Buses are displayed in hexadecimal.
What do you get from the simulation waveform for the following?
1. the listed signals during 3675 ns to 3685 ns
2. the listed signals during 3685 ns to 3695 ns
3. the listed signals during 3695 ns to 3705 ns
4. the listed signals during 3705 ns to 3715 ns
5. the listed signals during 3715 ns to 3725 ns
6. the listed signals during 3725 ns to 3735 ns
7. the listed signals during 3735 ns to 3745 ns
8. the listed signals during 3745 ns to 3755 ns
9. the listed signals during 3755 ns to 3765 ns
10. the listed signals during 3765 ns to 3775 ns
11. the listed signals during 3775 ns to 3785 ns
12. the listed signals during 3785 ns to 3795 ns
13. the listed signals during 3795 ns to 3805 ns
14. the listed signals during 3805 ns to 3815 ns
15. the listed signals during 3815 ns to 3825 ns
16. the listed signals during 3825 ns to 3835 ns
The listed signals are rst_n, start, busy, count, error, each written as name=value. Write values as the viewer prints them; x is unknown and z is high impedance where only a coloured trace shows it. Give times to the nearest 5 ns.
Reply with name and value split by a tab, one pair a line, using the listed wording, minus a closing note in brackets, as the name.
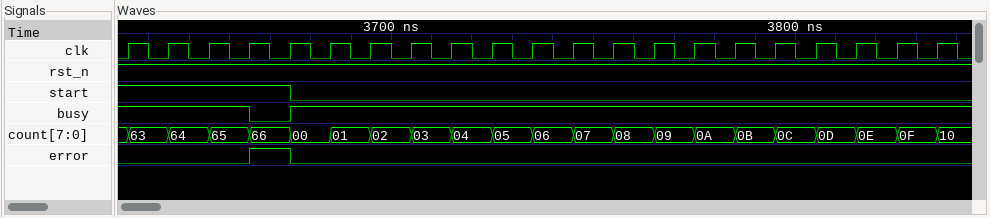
the listed signals during 3675 ns to 3685 ns	rst_n=1, start=0, busy=1, count=00, error=0
the listed signals during 3685 ns to 3695 ns	rst_n=1, start=0, busy=1, count=01, error=0
the listed signals during 3695 ns to 3705 ns	rst_n=1, start=0, busy=1, count=02, error=0
the listed signals during 3705 ns to 3715 ns	rst_n=1, start=0, busy=1, count=03, error=0
the listed signals during 3715 ns to 3725 ns	rst_n=1, start=0, busy=1, count=04, error=0
the listed signals during 3725 ns to 3735 ns	rst_n=1, start=0, busy=1, count=05, error=0
the listed signals during 3735 ns to 3745 ns	rst_n=1, start=0, busy=1, count=06, error=0
the listed signals during 3745 ns to 3755 ns	rst_n=1, start=0, busy=1, count=07, error=0
the listed signals during 3755 ns to 3765 ns	rst_n=1, start=0, busy=1, count=08, error=0
the listed signals during 3765 ns to 3775 ns	rst_n=1, start=0, busy=1, count=09, error=0
the listed signals during 3775 ns to 3785 ns	rst_n=1, start=0, busy=1, count=0A, error=0
the listed signals during 3785 ns to 3795 ns	rst_n=1, start=0, busy=1, count=0B, error=0
the listed signals during 3795 ns to 3805 ns	rst_n=1, start=0, busy=1, count=0C, error=0
the listed signals during 3805 ns to 3815 ns	rst_n=1, start=0, busy=1, count=0D, error=0
the listed signals during 3815 ns to 3825 ns	rst_n=1, start=0, busy=1, count=0E, error=0
the listed signals during 3825 ns to 3835 ns	rst_n=1, start=0, busy=1, count=0F, error=0
